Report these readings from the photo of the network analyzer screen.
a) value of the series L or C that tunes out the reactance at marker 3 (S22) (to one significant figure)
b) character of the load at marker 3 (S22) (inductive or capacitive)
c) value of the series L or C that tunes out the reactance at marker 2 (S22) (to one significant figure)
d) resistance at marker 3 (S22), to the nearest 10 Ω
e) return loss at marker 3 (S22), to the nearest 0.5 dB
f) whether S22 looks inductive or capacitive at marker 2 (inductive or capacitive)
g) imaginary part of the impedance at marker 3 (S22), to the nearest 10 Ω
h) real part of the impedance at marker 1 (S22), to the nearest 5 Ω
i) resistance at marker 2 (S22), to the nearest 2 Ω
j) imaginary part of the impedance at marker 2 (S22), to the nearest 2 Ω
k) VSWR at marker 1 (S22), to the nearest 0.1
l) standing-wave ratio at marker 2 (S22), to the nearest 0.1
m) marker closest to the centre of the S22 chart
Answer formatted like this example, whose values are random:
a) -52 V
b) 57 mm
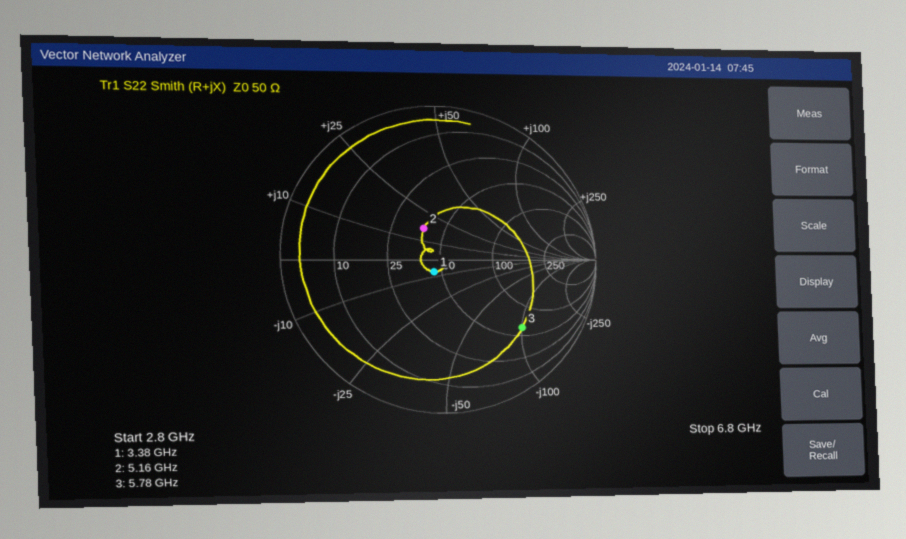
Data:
a) 3 nH
b) capacitive
c) 2 pF
d) 60 Ω
e) 3.5 dB
f) inductive
g) -100 Ω
h) 45 Ω
i) 38 Ω
j) +16 Ω
k) 1.2
l) 1.6
m) marker 1
